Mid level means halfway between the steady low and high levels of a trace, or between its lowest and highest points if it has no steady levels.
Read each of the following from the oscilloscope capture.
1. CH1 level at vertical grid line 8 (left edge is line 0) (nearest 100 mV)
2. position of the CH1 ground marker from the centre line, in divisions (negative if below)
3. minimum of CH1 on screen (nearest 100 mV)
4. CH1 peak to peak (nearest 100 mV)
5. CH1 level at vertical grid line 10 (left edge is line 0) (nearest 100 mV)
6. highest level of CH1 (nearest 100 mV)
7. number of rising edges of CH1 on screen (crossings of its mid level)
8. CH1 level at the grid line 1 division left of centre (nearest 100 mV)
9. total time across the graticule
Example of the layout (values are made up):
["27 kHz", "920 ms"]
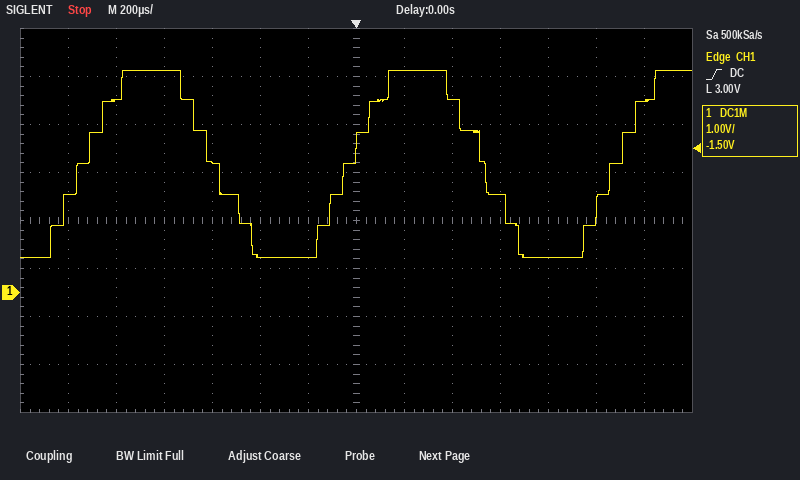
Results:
["4.6 V", "-1.5 div", "700 mV", "3.9 V", "2.0 V", "4.6 V", "3", "700 mV", "2.8 ms"]
